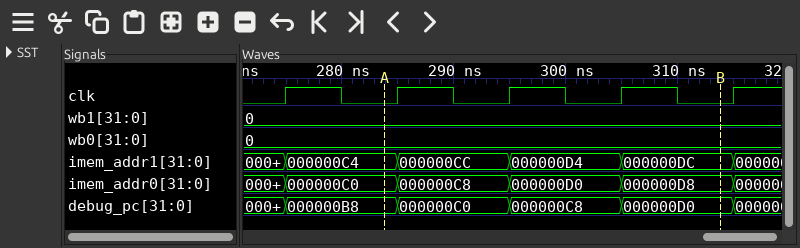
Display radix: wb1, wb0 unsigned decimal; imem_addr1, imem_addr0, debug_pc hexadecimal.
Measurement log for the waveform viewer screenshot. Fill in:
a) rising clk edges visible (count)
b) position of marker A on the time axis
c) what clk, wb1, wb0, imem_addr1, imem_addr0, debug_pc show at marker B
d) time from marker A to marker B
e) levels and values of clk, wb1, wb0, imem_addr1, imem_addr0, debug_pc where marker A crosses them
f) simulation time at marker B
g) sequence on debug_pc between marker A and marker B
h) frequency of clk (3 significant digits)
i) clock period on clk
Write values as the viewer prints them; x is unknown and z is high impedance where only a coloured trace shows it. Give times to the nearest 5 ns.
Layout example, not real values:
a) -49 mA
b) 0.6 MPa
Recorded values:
a) 5
b) 285 ns
c) clk=0, wb1=0, wb0=0, imem_addr1=000000DC, imem_addr0=000000D8, debug_pc=000000D0
d) 30 ns
e) clk=0, wb1=0, wb0=0, imem_addr1=000000C4, imem_addr0=000000C0, debug_pc=000000B8
f) 315 ns
g) 000000B8, 000000C0, 000000C8, 000000D0
h) 100 MHz
i) 10 ns
